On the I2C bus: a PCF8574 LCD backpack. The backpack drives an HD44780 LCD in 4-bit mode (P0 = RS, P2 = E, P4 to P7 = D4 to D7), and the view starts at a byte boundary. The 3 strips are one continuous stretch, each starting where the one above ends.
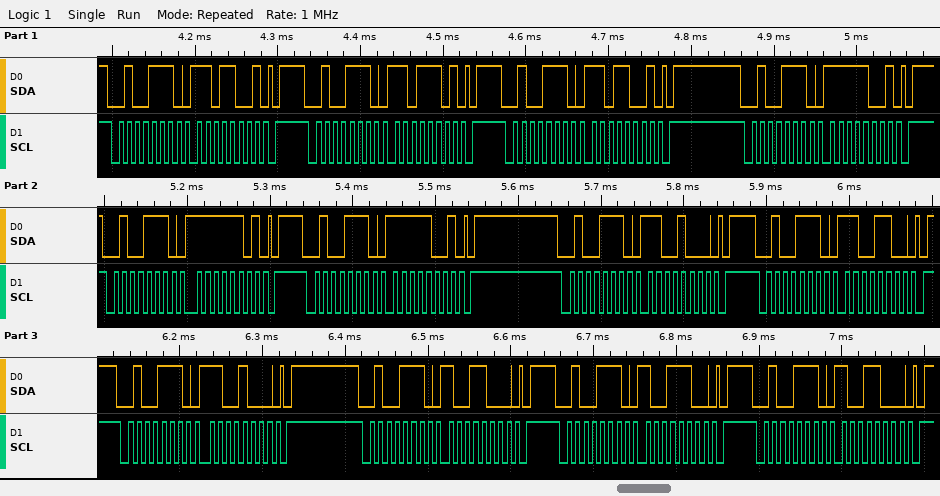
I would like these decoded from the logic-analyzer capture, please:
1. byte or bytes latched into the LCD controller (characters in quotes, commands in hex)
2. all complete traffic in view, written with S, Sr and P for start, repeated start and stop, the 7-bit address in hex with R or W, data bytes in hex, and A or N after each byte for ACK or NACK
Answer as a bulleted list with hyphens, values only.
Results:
- data 0xDF 0xC9
- S 27W A D9 A P S 27W A DD A P S 27W A D9 A P S 27W A F9 A P S 27W A FD A P S 27W A F9 A P S 27W A C8 A P S 27W A CC A P S 27W A C8 A P S 27W A 98 A P S 27W A 9C A P S 27W A 98 A P
